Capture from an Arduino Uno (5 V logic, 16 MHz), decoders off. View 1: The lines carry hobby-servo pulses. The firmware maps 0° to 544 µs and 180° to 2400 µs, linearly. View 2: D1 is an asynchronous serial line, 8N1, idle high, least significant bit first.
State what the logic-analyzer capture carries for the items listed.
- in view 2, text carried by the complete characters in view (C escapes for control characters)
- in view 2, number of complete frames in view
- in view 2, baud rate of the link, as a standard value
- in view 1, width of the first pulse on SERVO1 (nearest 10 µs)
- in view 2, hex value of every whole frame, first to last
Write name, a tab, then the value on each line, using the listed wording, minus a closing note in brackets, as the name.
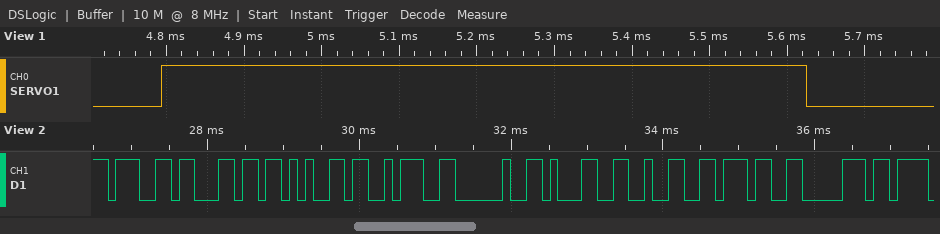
in view 2, text carried by the complete characters in view	"gle: 127p"
in view 2, number of complete frames in view	9
in view 2, baud rate of the link, as a standard value	9600 baud
in view 1, width of the first pulse on SERVO1	830 µs
in view 2, hex value of every whole frame, first to last	67 6C 65 3A 20 31 32 37 70
